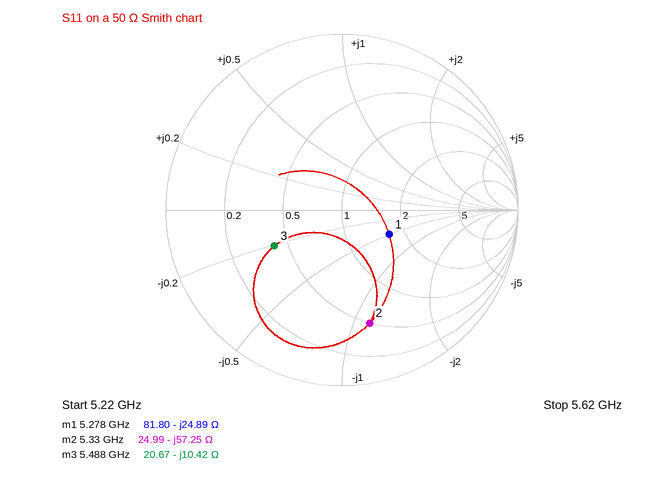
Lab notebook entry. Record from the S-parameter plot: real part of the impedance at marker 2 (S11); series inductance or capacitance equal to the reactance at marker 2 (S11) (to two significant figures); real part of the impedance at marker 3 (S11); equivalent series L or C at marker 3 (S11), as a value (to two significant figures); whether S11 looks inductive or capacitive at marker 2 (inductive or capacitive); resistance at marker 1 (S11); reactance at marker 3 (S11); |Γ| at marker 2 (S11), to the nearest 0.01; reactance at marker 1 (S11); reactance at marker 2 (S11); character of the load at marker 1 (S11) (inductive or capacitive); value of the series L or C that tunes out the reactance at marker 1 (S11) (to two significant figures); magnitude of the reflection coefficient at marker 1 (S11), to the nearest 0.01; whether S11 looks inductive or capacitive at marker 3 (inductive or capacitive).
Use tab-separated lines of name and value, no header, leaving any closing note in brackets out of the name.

real part of the impedance at marker 2	24.99 Ω
series inductance or capacitance equal to the reactance at marker 2 (S11)	520 fF
real part of the impedance at marker 3	20.67 Ω
equivalent series L or C at marker 3 (S11), as a value	2.8 pF
whether S11 looks inductive or capacitive at marker 2	capacitive
resistance at marker 1	81.80 Ω
reactance at marker 3	-10.42 Ω
|Γ| at marker 2 (S11), to the nearest 0.01	0.66
reactance at marker 1	-24.89 Ω
reactance at marker 2	-57.25 Ω
character of the load at marker 1 (S11)	capacitive
value of the series L or C that tunes out the reactance at marker 1 (S11)	750 pH
magnitude of the reflection coefficient at marker 1 (S11), to the nearest 0.01	0.30
whether S11 looks inductive or capacitive at marker 3	capacitive
